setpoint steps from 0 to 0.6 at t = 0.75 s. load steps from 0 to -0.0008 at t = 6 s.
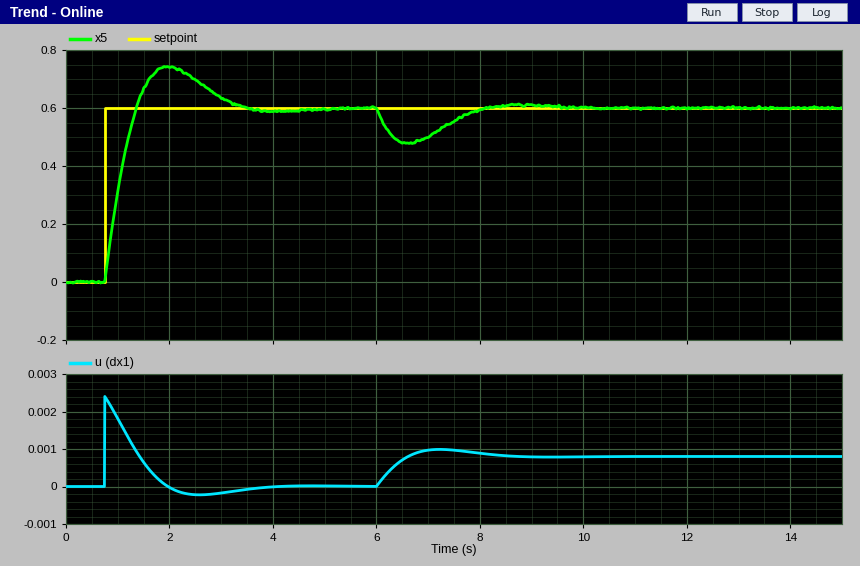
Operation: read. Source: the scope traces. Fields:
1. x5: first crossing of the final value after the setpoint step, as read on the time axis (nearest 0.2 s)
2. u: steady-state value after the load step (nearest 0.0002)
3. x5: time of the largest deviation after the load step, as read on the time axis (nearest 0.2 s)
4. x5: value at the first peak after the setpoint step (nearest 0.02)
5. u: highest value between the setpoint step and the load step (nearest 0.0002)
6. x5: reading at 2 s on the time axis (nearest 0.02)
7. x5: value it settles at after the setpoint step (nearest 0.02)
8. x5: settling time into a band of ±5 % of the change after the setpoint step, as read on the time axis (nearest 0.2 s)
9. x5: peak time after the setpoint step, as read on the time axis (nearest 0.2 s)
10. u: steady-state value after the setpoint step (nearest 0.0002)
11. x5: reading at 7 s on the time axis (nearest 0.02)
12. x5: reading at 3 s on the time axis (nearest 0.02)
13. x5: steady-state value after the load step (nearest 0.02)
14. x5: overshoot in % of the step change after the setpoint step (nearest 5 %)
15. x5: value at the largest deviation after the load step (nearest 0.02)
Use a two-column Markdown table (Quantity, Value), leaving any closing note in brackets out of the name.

| Quantity | Value |
|---|---|
| x5: first crossing of the final value after the setpoint step, as read on the time axis | 1.4 s |
| u: steady-state value after the load step | 0.0008 |
| x5: time of the largest deviation after the load step, as read on the time axis | 6.6 s |
| x5: value at the first peak after the setpoint step | 0.74 |
| u: highest value between the setpoint step and the load step | 0.0024 |
| x5: reading at 2 s on the time axis | 0.74 |
| x5: value it settles at after the setpoint step | 0.60 |
| x5: settling time into a band of ±5 % of the change after the setpoint step, as read on the time axis | 3.0 s |
| x5: peak time after the setpoint step, as read on the time axis | 2.0 s |
| u: steady-state value after the setpoint step | 0.0000 |
| x5: reading at 7 s on the time axis | 0.50 |
| x5: reading at 3 s on the time axis | 0.64 |
| x5: steady-state value after the load step | 0.60 |
| x5: overshoot in % of the step change after the setpoint step | 25 % |
| x5: value at the largest deviation after the load step | 0.48 |
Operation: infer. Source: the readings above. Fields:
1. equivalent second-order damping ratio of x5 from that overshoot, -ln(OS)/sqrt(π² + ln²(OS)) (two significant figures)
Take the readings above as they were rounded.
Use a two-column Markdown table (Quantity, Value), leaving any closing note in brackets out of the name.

| Quantity | Value |
|---|---|
| equivalent second-order damping ratio of x5 from that overshoot, -ln(OS)/sqrt(π² + ln²(OS)) | 0.40 |
